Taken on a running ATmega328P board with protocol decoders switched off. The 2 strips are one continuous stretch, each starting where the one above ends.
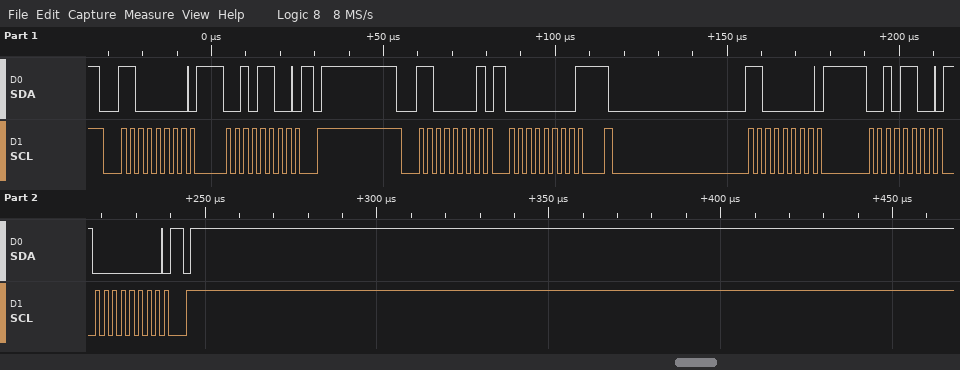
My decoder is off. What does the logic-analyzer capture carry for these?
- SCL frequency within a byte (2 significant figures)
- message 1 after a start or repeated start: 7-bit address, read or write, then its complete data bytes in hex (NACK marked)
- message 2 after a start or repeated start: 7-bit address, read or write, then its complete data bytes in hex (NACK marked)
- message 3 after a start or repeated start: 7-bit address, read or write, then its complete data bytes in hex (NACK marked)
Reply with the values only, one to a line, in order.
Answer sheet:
400 kHz
0x60 write: 2C
0x60 read: 00 NACK
0x60 write: 2C 00
